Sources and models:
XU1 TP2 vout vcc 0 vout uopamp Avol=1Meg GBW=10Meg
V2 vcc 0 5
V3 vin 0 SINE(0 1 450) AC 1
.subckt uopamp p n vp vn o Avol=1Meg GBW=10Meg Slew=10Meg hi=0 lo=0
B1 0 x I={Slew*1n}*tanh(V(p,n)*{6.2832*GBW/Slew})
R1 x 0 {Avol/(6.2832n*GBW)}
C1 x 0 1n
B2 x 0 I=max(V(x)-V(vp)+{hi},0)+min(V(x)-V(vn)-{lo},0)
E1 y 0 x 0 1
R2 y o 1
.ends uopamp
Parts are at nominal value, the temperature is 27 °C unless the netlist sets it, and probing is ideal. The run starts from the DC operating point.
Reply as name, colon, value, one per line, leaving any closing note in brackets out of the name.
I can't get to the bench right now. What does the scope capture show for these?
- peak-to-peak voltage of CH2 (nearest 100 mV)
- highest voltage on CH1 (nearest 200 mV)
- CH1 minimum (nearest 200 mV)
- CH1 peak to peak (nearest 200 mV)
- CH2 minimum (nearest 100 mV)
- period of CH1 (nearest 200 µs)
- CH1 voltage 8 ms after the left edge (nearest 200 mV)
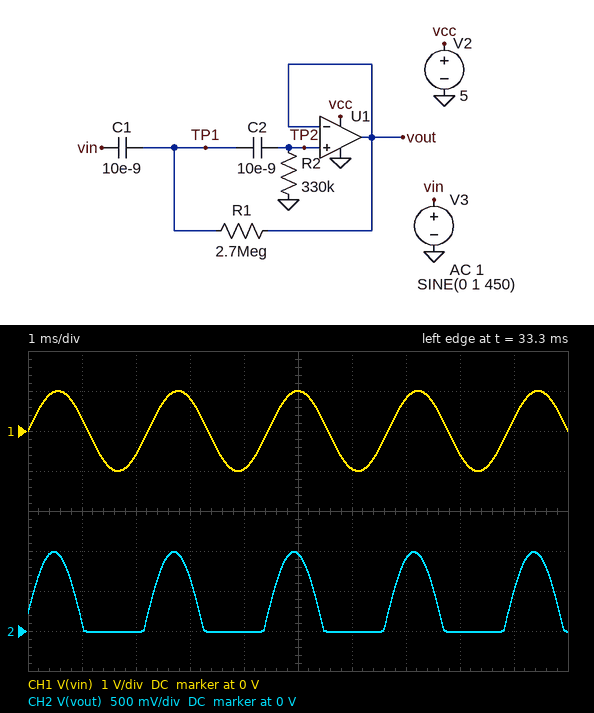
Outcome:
peak-to-peak voltage of CH2: 1.0 V
highest voltage on CH1: 1.0 V
CH1 minimum: -1.0 V
CH1 peak to peak: 2.0 V
CH2 minimum: 0 V
period of CH1: 2.2 ms
CH1 voltage 8 ms after the left edge: -600 mV
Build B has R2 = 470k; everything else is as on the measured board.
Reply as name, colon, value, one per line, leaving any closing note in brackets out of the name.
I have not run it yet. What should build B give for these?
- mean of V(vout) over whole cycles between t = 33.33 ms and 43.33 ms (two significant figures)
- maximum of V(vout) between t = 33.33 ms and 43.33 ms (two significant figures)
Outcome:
mean of V(vout) over whole cycles between t = 33.33 ms and 43.33 ms: 320 mV
maximum of V(vout) between t = 33.33 ms and 43.33 ms: 1.0 V
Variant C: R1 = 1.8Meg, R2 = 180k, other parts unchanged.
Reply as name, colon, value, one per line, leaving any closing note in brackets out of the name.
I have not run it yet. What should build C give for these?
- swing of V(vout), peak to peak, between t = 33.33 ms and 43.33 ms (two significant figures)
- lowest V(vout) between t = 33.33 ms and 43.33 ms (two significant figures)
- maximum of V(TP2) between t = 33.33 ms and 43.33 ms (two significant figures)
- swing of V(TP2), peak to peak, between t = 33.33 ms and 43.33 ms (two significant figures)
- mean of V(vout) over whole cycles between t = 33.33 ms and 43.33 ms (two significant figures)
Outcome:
swing of V(vout), peak to peak, between t = 33.33 ms and 43.33 ms: 950 mV
lowest V(vout) between t = 33.33 ms and 43.33 ms: -10 mV
maximum of V(TP2) between t = 33.33 ms and 43.33 ms: 940 mV
swing of V(TP2), peak to peak, between t = 33.33 ms and 43.33 ms: 1.9 V
mean of V(vout) over whole cycles between t = 33.33 ms and 43.33 ms: 290 mV
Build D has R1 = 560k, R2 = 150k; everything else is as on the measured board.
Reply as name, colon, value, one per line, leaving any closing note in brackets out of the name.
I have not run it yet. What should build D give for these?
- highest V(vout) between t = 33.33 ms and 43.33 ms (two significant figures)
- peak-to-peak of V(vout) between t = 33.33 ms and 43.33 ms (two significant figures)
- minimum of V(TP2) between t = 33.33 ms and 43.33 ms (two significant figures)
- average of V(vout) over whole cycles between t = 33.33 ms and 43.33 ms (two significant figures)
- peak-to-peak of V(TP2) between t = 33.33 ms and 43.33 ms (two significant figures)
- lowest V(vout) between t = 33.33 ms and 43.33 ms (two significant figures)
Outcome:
highest V(vout) between t = 33.33 ms and 43.33 ms: 910 mV
peak-to-peak of V(vout) between t = 33.33 ms and 43.33 ms: 920 mV
minimum of V(TP2) between t = 33.33 ms and 43.33 ms: -900 mV
average of V(vout) over whole cycles between t = 33.33 ms and 43.33 ms: 280 mV
peak-to-peak of V(TP2) between t = 33.33 ms and 43.33 ms: 1.8 V
lowest V(vout) between t = 33.33 ms and 43.33 ms: -10 mV
